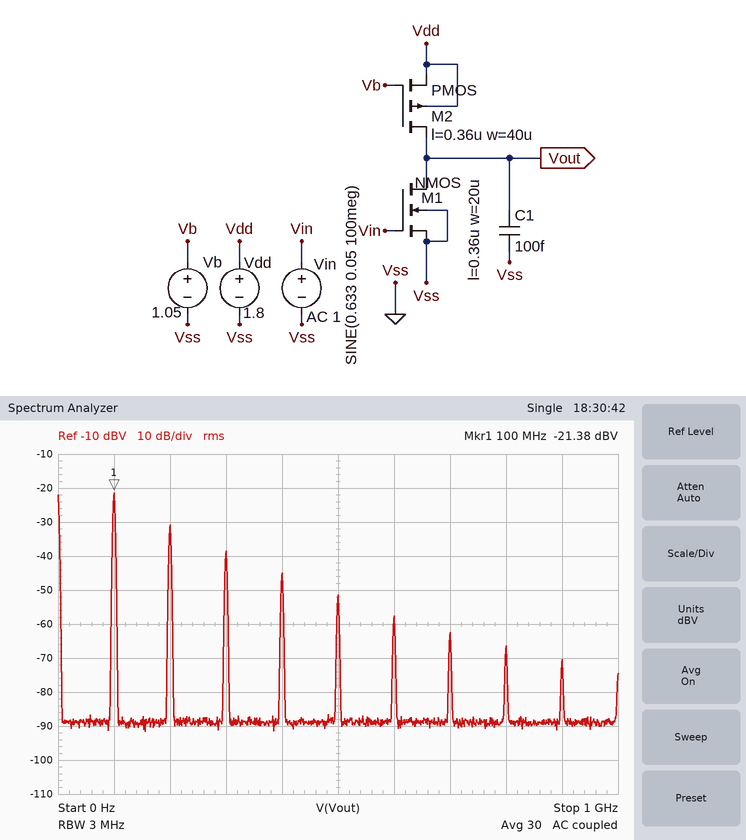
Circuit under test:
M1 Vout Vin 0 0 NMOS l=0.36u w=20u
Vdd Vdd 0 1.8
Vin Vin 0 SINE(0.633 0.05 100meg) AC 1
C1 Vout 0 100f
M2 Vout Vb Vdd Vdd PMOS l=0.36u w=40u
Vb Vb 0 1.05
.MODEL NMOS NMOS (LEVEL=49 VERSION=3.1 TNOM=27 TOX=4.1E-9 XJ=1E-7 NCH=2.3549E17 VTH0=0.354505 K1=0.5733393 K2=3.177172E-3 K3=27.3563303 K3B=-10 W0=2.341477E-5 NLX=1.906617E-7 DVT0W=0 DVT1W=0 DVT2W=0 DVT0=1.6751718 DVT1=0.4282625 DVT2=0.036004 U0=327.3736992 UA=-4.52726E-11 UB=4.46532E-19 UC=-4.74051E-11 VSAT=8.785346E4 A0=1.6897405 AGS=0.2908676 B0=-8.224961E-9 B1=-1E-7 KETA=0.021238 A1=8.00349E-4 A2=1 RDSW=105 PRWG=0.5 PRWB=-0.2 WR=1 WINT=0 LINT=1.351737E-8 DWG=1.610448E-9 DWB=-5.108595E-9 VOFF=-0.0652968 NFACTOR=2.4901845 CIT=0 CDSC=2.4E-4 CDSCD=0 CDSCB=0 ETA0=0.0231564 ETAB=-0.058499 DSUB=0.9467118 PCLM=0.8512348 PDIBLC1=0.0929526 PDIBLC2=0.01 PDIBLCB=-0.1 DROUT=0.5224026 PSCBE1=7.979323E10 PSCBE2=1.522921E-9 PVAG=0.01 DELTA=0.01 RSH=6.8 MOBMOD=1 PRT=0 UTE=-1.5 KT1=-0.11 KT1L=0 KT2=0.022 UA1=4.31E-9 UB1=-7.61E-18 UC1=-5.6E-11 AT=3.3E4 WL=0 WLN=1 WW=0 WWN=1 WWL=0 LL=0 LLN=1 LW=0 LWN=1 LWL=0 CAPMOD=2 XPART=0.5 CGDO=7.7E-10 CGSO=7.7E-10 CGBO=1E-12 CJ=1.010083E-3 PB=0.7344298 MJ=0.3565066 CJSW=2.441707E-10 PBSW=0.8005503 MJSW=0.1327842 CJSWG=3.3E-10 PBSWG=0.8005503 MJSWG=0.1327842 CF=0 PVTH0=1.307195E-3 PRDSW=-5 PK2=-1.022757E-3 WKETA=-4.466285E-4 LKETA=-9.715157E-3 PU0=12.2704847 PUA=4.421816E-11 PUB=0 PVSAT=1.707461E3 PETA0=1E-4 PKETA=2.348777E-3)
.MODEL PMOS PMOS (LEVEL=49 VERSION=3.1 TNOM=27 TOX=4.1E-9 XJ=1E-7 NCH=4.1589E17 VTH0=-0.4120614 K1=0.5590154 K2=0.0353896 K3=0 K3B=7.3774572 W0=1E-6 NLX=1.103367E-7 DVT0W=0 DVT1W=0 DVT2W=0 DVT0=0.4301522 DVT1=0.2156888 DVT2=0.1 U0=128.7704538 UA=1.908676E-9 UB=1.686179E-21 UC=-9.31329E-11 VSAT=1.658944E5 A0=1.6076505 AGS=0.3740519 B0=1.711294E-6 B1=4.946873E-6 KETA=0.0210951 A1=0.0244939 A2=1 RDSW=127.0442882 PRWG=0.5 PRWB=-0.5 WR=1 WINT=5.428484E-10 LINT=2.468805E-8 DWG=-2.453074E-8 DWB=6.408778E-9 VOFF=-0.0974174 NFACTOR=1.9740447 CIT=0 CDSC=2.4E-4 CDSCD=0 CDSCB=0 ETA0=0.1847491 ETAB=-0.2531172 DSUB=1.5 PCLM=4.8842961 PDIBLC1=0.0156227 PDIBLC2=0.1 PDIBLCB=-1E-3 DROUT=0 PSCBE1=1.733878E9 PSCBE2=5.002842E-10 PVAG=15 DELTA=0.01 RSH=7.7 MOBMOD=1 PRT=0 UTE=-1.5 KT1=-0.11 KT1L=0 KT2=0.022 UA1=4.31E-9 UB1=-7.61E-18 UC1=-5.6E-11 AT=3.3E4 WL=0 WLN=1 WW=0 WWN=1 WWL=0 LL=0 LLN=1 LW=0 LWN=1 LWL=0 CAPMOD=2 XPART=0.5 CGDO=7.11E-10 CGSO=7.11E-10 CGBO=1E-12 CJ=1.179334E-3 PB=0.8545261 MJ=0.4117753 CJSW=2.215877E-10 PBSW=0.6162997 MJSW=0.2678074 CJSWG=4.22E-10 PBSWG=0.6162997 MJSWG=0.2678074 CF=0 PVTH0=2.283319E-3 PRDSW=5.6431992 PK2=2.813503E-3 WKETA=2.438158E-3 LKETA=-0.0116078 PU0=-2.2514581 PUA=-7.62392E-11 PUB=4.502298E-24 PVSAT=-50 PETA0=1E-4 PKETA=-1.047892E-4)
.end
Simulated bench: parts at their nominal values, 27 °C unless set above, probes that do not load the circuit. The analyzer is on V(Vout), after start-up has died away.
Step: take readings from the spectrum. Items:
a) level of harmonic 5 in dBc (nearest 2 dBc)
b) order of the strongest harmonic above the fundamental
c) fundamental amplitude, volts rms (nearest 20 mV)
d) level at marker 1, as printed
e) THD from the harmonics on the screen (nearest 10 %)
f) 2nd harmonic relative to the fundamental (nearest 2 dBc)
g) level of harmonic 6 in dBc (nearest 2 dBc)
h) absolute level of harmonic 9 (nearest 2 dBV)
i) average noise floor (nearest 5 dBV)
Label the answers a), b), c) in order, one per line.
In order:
a) -30 dBc
b) 2
c) 80 mV
d) -21.38 dBV
e) 40 %
f) -10 dBc
g) -36 dBc
h) -70 dBV
i) -90 dBV
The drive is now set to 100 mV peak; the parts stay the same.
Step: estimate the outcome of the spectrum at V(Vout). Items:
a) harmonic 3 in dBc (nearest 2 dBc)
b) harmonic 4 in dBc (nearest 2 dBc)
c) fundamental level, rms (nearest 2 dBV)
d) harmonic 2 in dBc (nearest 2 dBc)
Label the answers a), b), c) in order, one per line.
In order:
a) -22 dBc
b) -26 dBc
c) -6 dBV
d) -8 dBc
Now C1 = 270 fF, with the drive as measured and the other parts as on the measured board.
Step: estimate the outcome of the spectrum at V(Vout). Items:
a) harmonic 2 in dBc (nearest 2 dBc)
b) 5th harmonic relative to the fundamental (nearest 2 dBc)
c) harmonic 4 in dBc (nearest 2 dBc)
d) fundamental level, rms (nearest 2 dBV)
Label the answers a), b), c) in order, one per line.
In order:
a) -12 dBc
b) -38 dBc
c) -30 dBc
d) -22 dBV
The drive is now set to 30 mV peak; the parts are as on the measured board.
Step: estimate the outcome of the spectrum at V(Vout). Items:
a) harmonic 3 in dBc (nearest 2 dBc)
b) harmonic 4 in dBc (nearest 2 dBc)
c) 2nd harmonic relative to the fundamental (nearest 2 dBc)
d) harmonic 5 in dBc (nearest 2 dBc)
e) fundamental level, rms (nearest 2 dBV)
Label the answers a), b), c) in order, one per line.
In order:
a) -32 dBc
b) -44 dBc
c) -16 dBc
d) -56 dBc
e) -28 dBV
